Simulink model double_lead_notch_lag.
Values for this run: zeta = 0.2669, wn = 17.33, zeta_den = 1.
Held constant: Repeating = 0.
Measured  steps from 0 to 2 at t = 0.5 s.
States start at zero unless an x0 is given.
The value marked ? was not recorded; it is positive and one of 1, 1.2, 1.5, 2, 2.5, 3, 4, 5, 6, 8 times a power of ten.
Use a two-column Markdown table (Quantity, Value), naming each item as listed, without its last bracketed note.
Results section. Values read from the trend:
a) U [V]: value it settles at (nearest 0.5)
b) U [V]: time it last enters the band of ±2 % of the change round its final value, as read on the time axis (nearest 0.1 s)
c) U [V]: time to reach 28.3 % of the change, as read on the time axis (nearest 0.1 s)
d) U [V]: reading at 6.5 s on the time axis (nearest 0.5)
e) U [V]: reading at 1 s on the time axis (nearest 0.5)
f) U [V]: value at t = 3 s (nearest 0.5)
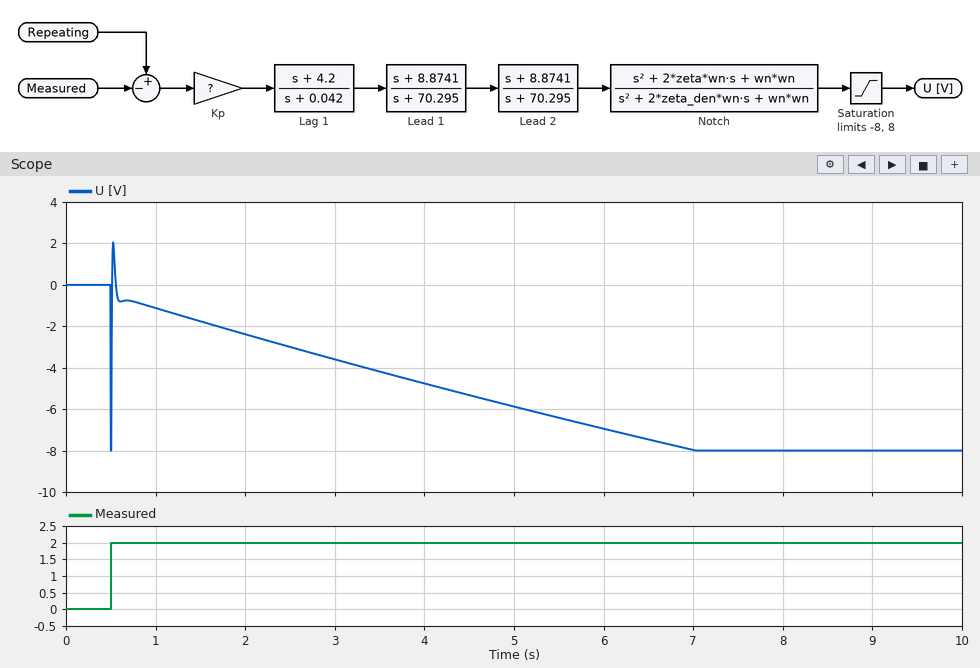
| Quantity | Value |
|---|---|
| U [V]: value it settles at | -8.0 |
| U [V]: time it last enters the band of ±2 % of the change round its final value, as read on the time axis | 6.9 s |
| U [V]: time to reach 28.3 % of the change, as read on the time axis | 0.5 s |
| U [V]: reading at 6.5 s on the time axis | -7.5 |
| U [V]: reading at 1 s on the time axis | -1.0 |
| U [V]: value at t = 3 s | -3.5 |
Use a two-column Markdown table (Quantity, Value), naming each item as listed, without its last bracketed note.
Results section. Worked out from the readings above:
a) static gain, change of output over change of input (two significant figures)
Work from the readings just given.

| Quantity | Value |
|---|---|
| static gain, change of output over change of input | -4.0 |
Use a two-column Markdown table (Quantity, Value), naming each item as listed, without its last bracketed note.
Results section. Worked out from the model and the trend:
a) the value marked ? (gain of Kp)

| Quantity | Value |
|---|---|
| the value marked ? | 10 |
